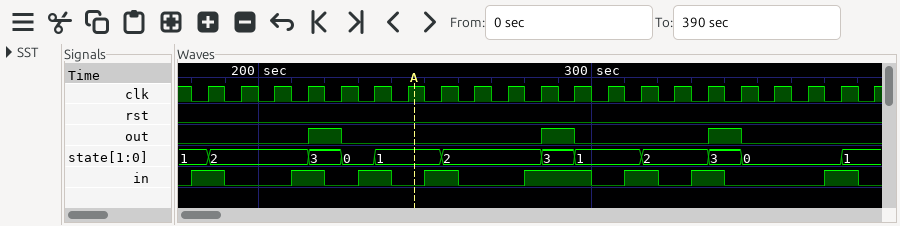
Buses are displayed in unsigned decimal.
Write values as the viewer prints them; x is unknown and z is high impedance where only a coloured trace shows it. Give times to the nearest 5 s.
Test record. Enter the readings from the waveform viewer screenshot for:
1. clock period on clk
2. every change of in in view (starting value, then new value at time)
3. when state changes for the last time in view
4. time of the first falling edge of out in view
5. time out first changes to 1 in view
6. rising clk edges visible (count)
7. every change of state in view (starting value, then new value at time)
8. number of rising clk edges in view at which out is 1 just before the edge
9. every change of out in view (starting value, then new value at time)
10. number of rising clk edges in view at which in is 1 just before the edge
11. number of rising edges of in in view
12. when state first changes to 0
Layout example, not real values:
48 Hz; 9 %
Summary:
10 s; 0, 1 at 180 s, 0 at 190 s, 1 at 210 s, 0 at 220 s, 1 at 230 s, 0 at 240 s, 1 at 250 s, 0 at 260 s, 1 at 280 s, 0 at 300 s, 1 at 310 s, 0 at 320 s, 1 at 330 s, 0 at 340 s, 1 at 370 s, 0 at 380 s; 375 s; 225 s; 215 s; 21; 1, 2 at 185 s, 3 at 215 s, 0 at 225 s, 1 at 235 s, 2 at 255 s, 3 at 285 s, 1 at 295 s, 2 at 315 s, 3 at 335 s, 0 at 345 s, 1 at 375 s; 3; 0, 1 at 215 s, 0 at 225 s, 1 at 285 s, 0 at 295 s, 1 at 335 s, 0 at 345 s; 9; 8; 225 s
